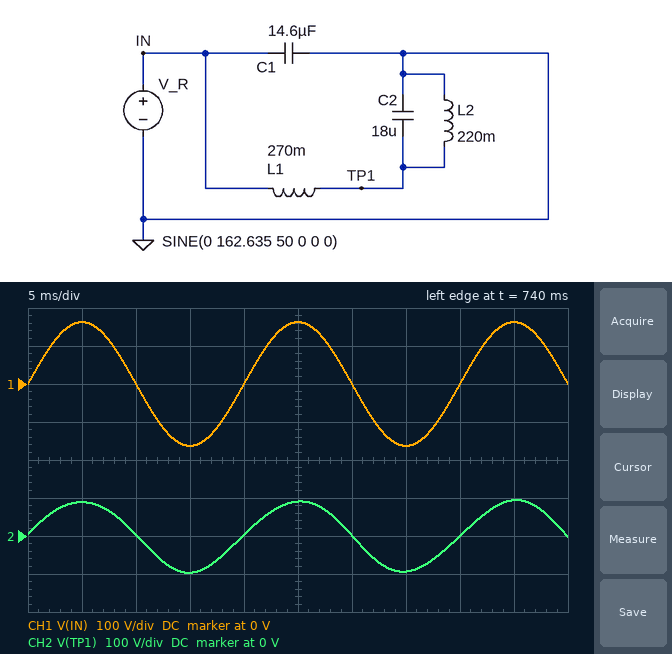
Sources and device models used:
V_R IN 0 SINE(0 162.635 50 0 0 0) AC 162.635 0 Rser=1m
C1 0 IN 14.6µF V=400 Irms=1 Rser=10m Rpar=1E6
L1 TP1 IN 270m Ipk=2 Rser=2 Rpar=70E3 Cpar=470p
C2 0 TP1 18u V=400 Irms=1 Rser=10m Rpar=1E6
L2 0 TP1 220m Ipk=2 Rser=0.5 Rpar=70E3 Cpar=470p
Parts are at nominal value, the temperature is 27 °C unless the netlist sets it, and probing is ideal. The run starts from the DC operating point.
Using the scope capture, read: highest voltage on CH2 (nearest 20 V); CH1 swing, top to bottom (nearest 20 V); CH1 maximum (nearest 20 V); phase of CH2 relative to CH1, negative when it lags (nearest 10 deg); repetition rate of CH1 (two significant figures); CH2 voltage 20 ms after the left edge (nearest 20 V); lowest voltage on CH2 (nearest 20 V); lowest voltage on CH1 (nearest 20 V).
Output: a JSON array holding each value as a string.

["100 V", "320 V", "160 V", "0 deg", "50 Hz", "0 V", "-100 V", "-160 V"]
